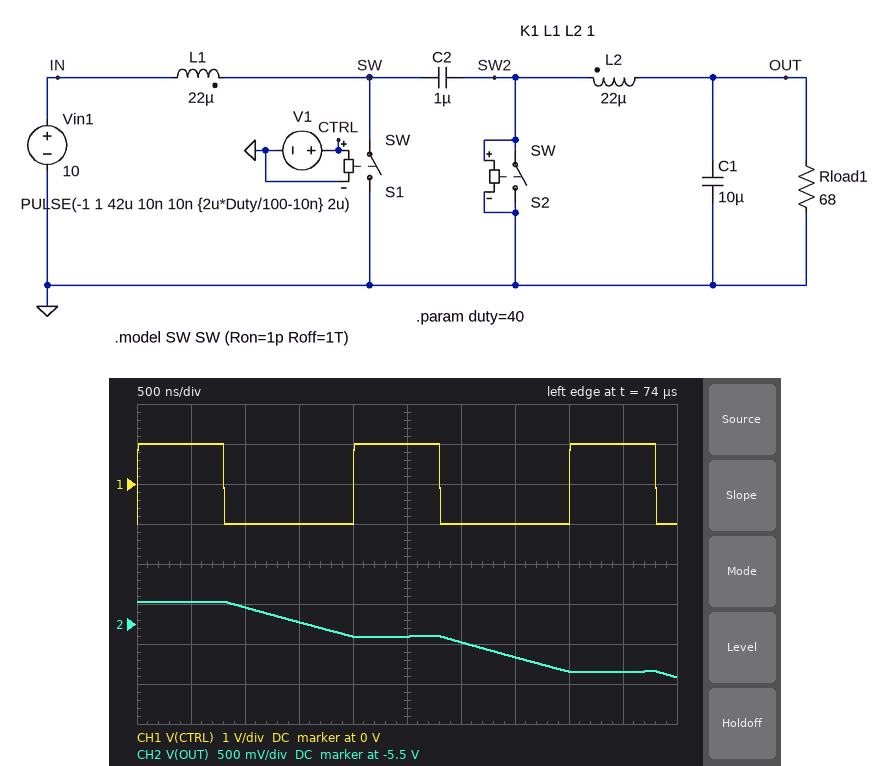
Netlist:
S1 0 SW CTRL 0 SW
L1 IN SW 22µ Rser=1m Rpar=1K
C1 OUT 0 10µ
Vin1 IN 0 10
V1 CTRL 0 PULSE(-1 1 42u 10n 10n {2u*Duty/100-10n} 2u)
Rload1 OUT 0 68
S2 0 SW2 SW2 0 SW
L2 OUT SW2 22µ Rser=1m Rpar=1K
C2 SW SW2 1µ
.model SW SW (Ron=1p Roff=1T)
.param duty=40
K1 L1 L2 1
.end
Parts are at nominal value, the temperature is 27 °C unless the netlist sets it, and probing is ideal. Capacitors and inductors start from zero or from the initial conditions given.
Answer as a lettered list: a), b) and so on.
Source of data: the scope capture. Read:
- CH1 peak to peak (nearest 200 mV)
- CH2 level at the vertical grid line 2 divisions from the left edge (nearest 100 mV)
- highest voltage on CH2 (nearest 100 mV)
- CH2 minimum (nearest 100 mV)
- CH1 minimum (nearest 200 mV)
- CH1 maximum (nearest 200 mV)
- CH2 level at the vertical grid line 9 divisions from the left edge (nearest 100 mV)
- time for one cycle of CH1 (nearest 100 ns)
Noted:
a) 2.0 V
b) -5.3 V
c) -5.2 V
d) -6.2 V
e) -1.0 V
f) 1.0 V
g) -6.1 V
h) 2.0 µs
